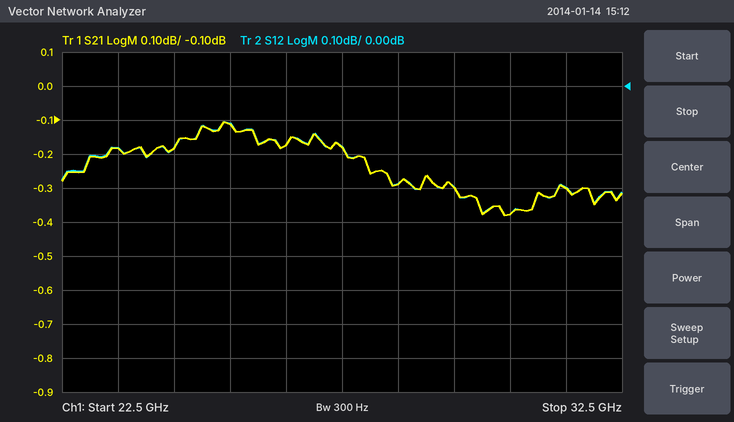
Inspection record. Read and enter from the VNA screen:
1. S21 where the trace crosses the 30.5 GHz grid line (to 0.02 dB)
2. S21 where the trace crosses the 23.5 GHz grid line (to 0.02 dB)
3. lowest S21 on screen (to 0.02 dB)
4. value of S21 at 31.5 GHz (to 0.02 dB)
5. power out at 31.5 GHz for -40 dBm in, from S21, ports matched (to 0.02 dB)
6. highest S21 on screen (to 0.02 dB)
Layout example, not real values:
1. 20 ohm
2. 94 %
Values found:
1. -0.38 dB
2. -0.18 dB
3. -0.38 dB
4. -0.30 dB
5. -40.30 dBm
6. -0.10 dB
